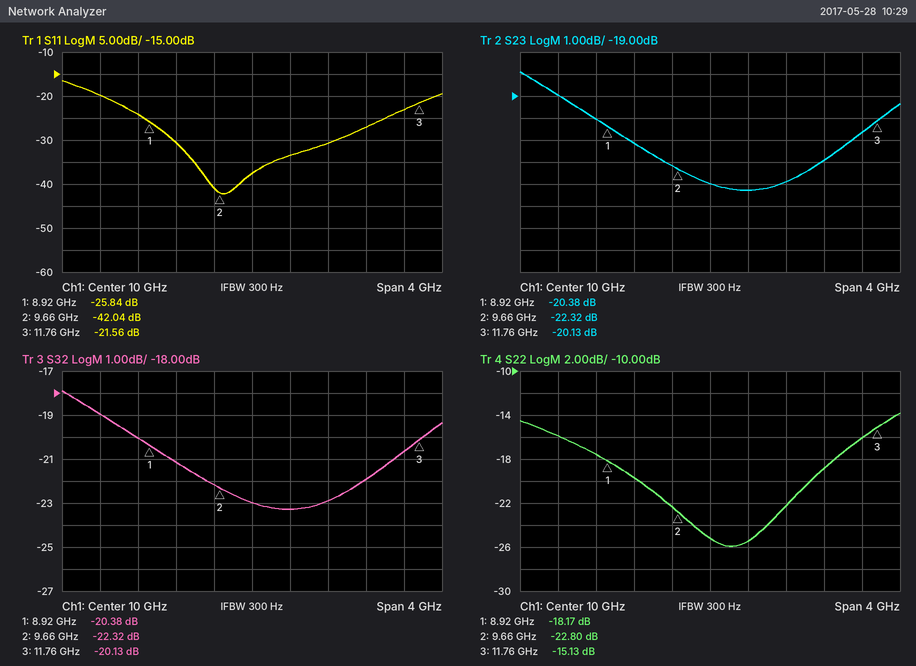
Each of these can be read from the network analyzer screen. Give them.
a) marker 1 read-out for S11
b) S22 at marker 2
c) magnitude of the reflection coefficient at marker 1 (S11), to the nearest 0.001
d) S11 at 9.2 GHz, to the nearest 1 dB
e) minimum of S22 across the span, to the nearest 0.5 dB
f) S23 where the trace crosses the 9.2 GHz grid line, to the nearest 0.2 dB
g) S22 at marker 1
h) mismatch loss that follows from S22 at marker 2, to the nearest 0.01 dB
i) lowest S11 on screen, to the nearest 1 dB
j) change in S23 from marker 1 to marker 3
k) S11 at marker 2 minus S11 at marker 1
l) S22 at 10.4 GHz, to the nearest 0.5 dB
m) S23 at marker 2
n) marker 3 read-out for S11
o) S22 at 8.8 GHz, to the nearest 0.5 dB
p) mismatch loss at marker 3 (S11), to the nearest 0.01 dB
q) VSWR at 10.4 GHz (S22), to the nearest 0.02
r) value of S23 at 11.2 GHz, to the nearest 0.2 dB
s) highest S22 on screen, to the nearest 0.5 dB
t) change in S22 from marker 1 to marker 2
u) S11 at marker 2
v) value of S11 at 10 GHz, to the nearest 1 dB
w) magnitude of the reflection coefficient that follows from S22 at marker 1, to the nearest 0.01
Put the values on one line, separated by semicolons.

-25.84 dB; -22.80 dB; 0.051; -31 dB; -26.0 dB; -21.2 dB; -18.17 dB; 0.02 dB; -42 dB; 0.25 dB; -16.20 dB; -25.5 dB; -22.32 dB; -21.56 dB; -17.5 dB; 0.03 dB; 1.12; -22.0 dB; -14.0 dB; -4.63 dB; -42.04 dB; -38 dB; 0.12
